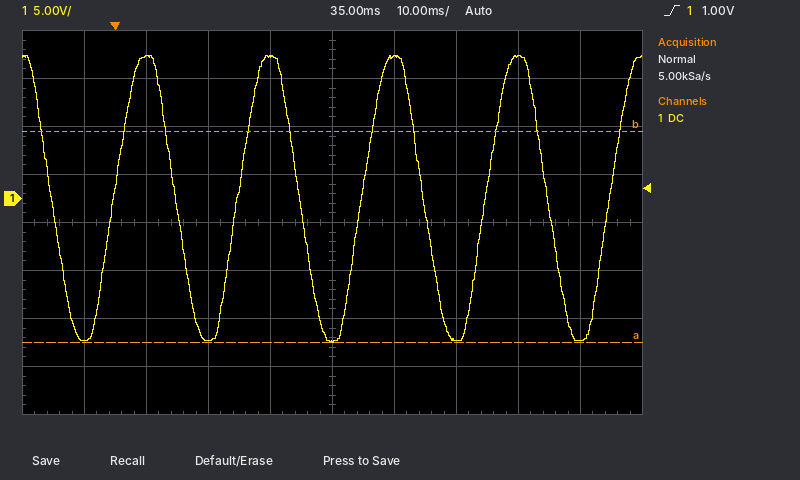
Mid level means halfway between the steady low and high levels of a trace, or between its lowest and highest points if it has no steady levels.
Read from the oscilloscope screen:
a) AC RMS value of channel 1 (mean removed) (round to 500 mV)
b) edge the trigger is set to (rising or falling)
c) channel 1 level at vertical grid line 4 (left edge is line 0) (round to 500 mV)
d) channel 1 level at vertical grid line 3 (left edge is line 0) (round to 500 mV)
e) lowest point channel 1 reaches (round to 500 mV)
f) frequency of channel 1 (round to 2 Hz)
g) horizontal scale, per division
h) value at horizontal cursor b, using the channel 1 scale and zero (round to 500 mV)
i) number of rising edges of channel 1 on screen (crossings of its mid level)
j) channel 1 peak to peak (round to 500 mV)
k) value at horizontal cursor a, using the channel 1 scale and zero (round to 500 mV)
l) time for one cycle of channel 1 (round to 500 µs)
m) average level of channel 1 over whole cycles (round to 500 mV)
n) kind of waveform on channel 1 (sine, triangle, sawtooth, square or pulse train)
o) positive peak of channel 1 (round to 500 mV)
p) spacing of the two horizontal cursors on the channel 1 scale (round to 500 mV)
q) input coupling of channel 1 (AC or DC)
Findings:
10.5 V
rising
15.0 V
-15.0 V
-15.0 V
50 Hz
10 ms
7.0 V
5
30.0 V
-15.0 V
20.0 ms
0.0 V
sine
15.0 V
22.0 V
DC
